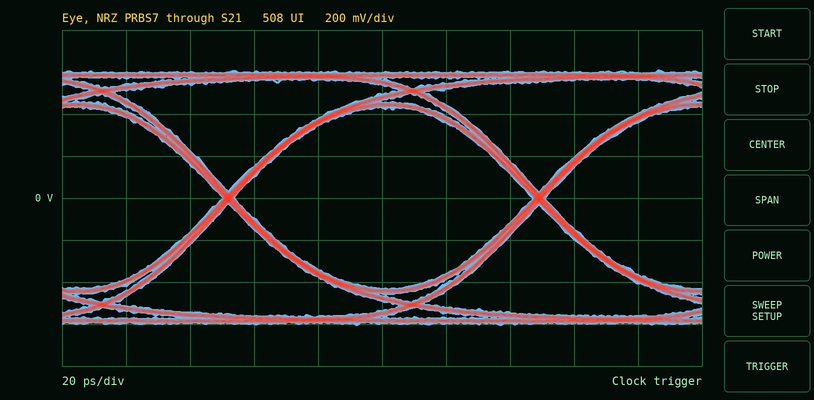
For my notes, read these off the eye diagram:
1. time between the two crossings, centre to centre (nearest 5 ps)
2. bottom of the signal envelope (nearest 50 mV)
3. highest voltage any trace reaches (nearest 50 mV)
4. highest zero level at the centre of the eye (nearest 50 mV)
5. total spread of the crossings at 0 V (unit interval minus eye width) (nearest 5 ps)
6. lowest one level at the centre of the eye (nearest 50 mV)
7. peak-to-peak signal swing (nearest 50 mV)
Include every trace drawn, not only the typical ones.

95 ps
-600 mV
600 mV
-450 mV
5 ps
450 mV
1.20 V
